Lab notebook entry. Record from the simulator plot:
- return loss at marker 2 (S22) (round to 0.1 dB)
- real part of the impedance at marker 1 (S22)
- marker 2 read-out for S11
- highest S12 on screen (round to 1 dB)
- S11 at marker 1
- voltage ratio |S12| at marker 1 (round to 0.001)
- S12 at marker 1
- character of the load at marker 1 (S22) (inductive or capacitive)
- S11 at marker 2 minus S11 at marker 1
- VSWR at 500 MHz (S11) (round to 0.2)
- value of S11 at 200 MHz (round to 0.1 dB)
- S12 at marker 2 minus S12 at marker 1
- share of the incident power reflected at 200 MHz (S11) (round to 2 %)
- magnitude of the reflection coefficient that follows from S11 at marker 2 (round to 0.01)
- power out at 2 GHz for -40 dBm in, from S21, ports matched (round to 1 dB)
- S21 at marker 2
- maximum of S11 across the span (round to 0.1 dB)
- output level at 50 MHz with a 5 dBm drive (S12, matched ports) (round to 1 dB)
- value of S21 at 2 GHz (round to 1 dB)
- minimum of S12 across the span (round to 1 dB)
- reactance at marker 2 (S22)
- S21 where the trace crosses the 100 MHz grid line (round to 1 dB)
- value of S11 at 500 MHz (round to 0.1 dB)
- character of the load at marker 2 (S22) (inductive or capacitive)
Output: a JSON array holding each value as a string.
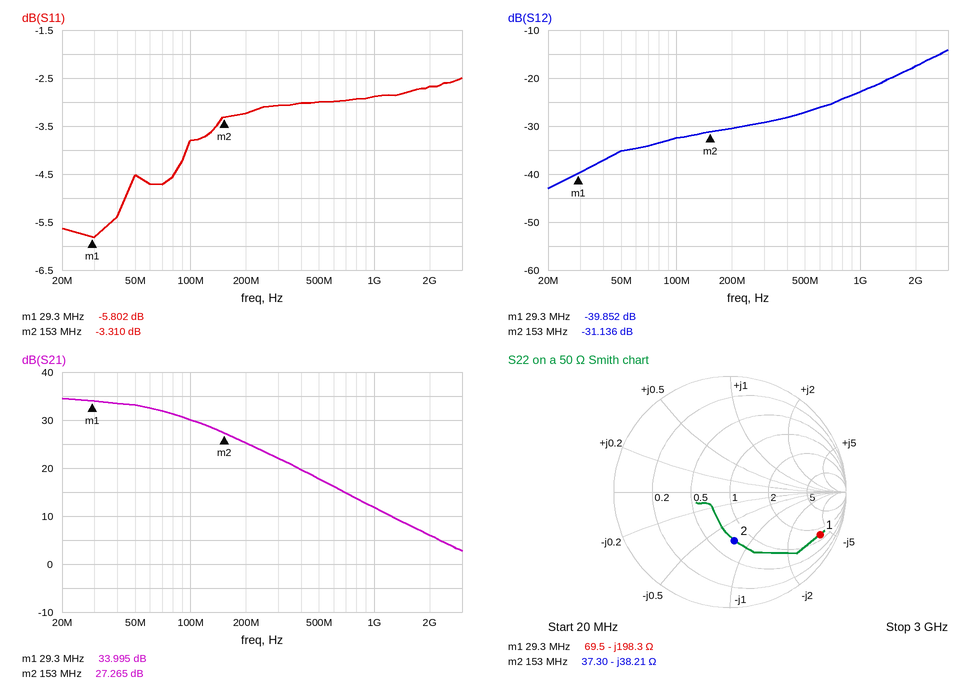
["7.5 dB", "69.5 Ω", "-3.310 dB", "-14 dB", "-5.802 dB", "0.010", "-39.852 dB", "capacitive", "2.492 dB", "5.8", "-3.2 dB", "8.716 dB", "48 %", "0.68", "-34 dBm", "27.265 dB", "-2.5 dB", "-30 dBm", "6 dB", "-43 dB", "-38.21 Ω", "30 dB", "-3.0 dB", "capacitive"]
